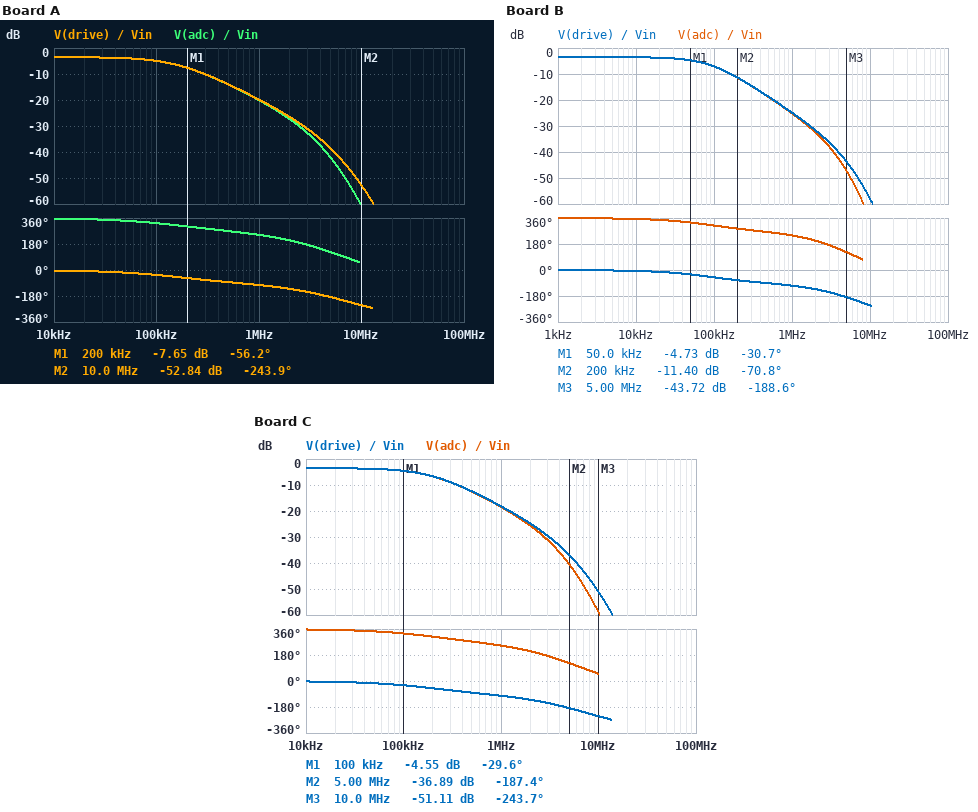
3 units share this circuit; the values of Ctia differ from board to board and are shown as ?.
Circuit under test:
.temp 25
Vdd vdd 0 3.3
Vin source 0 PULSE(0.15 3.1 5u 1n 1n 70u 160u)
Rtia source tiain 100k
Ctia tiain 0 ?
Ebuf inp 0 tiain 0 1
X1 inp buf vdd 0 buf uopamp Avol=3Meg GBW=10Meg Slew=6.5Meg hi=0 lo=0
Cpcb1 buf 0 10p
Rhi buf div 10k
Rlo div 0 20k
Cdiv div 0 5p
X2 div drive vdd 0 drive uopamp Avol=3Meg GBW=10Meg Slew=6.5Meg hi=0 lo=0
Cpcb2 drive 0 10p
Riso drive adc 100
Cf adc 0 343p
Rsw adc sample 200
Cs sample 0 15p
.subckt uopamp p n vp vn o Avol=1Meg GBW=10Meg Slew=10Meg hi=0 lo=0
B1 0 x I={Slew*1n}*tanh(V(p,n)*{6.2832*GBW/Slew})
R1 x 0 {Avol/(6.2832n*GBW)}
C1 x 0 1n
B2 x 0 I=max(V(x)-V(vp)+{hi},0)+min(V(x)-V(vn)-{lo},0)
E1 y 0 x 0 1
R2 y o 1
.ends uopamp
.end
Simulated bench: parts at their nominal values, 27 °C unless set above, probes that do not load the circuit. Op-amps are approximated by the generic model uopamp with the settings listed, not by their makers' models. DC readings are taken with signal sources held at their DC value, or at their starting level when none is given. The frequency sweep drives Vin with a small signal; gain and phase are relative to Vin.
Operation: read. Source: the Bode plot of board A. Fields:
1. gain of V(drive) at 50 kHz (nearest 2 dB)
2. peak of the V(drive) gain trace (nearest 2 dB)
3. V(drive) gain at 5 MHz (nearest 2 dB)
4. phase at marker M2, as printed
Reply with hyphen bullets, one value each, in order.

- -4 dB
- -4 dB
- -38 dB
- -243.9 deg
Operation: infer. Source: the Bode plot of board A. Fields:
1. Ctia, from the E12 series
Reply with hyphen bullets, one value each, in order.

- 10 pF
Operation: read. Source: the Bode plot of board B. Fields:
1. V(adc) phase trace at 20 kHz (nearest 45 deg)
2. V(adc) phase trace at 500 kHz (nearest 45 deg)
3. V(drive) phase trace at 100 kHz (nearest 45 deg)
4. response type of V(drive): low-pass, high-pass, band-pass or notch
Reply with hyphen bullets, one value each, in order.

- 360 deg
- 270 deg
- -45 deg
- low-pass
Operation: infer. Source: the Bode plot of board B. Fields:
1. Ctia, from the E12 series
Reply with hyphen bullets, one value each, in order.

- 18 pF
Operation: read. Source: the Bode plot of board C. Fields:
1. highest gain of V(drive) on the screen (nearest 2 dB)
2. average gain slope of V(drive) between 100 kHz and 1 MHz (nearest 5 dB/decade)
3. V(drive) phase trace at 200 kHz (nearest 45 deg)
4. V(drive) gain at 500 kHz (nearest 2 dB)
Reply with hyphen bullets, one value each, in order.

- -4 dB
- -15 dB/decade
- -45 deg
- -12 dB
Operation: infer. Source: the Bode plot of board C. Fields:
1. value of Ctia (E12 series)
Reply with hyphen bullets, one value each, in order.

- 8.2 pF
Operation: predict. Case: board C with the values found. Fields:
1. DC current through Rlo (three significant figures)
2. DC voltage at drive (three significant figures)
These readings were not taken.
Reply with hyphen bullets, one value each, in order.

- 5.00 µA
- 100 mV
